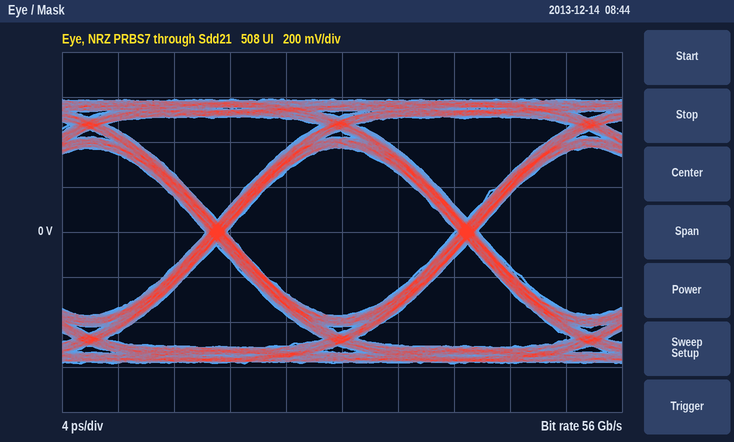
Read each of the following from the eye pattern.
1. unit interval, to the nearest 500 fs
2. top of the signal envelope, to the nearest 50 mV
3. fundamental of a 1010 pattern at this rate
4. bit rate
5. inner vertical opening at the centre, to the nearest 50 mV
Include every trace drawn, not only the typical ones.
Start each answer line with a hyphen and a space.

- 18.0 ps
- 600 mV
- 28 GHz
- 56 Gb/s
- 750 mV
